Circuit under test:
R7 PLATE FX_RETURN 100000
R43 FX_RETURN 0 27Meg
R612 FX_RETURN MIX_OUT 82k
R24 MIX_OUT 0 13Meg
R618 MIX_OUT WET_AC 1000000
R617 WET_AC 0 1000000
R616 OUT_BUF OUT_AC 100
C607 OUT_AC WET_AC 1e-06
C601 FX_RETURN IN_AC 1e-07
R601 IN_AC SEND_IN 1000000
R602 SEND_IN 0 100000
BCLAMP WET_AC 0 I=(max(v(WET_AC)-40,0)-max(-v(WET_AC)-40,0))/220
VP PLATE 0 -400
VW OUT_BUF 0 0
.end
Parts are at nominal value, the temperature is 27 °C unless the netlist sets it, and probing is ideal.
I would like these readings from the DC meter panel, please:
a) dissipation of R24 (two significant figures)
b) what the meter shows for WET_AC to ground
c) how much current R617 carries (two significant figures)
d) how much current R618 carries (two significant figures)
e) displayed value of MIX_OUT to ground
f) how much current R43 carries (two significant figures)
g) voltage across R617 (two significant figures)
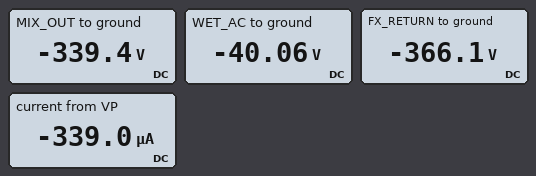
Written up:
8.9 mW
-40.06 V
40 µA
300 µA
-339.4 V
14 µA
40 V
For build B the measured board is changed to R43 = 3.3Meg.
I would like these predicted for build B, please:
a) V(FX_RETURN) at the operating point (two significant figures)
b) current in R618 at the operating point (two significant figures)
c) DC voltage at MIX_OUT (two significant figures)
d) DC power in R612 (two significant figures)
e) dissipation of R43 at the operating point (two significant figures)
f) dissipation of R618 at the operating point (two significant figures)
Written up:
-360 V
290 µA
-330 V
8.2 mW
39 mW
85 mW
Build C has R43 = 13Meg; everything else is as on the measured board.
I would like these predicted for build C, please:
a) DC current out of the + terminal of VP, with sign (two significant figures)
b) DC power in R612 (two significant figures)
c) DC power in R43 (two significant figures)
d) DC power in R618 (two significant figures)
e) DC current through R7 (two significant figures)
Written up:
-350 µA
8.6 mW
10 mW
89 mW
350 µA
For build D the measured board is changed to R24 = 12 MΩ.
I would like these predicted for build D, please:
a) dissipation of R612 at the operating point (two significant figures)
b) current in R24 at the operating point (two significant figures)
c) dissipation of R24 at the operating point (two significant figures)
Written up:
8.8 mW
28 µA
9.6 mW
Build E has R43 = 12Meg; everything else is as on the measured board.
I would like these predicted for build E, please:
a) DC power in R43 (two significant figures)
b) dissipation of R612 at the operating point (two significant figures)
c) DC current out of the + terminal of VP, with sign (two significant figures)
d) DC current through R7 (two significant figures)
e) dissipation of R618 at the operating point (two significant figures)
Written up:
11 mW
8.6 mW
-350 µA
350 µA
89 mW
